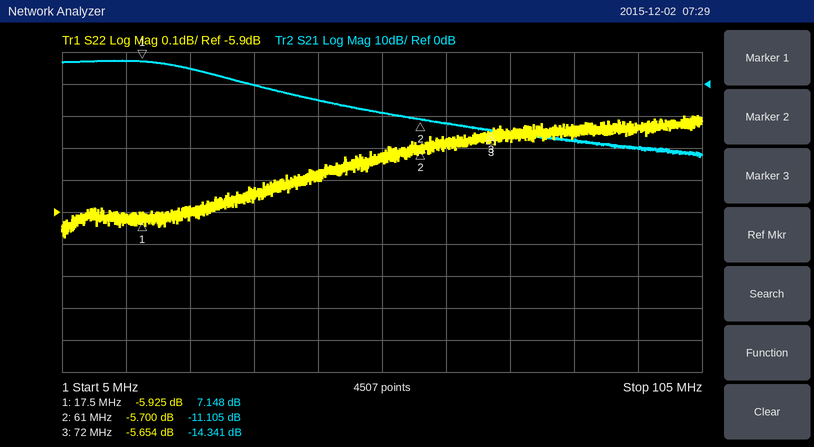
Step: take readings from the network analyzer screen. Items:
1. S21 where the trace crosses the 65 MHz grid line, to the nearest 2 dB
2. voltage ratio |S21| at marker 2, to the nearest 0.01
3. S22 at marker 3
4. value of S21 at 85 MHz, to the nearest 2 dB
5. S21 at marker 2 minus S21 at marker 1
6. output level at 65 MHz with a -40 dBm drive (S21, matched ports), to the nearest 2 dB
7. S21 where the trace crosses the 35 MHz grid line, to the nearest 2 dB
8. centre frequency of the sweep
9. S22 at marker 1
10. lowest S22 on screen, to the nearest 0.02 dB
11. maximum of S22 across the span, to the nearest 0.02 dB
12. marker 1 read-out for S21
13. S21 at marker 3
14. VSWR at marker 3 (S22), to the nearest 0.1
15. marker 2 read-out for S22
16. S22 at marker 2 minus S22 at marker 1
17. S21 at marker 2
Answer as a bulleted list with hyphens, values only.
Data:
- -12 dB
- 0.28
- -5.654 dB
- -18 dB
- -18.253 dB
- -52 dBm
- 0 dB
- 55 MHz
- -5.925 dB
- -5.98 dB
- -5.60 dB
- 7.148 dB
- -14.341 dB
- 3.2
- -5.700 dB
- 0.225 dB
- -11.105 dB
